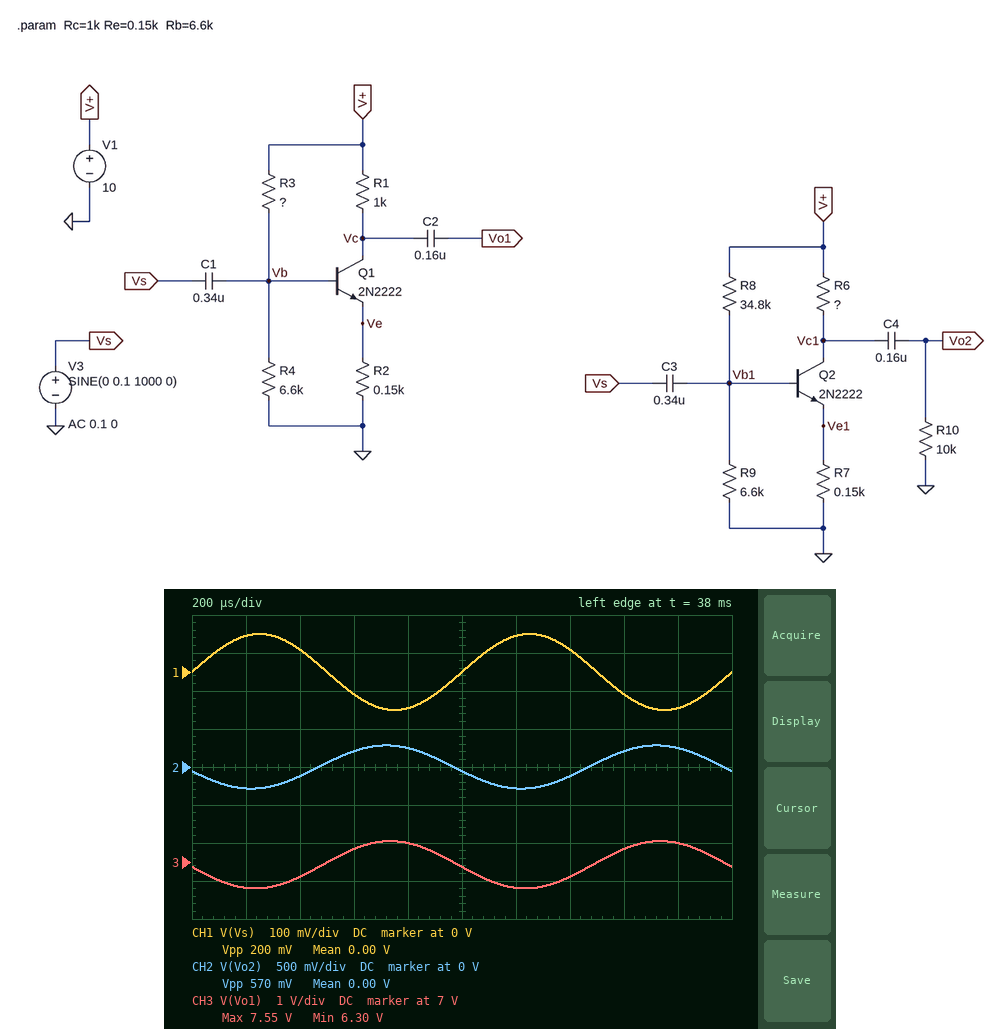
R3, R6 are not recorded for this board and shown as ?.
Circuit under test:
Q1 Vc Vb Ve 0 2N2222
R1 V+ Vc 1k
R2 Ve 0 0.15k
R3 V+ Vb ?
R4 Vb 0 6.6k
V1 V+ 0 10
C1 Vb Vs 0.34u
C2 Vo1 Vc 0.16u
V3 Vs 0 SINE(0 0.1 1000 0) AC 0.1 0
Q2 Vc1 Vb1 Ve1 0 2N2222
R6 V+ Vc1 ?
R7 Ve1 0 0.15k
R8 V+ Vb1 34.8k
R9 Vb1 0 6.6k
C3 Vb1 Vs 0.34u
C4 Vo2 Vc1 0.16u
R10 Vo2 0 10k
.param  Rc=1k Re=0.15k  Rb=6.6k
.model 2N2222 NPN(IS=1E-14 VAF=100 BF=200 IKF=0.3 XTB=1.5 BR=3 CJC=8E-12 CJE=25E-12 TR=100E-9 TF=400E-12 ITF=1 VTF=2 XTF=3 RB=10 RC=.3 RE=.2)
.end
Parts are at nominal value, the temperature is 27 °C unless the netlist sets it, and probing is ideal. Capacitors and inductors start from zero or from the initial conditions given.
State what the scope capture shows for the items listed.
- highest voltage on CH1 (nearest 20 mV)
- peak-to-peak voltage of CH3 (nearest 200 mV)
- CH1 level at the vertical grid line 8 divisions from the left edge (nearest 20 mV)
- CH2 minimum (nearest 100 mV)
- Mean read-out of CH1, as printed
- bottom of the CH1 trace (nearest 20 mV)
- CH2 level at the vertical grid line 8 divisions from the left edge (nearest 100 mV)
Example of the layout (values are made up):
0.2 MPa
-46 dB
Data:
100 mV
1.2 V
-60 mV
-300 mV
0.00 V
-100 mV
200 mV
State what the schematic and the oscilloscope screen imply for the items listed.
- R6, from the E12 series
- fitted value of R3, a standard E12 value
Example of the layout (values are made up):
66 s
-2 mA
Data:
470 Ω
47 kΩ
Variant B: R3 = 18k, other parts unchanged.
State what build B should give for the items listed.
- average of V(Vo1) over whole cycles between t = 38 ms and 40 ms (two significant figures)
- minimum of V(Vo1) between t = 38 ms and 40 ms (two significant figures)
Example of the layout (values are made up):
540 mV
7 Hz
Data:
1.5 V
1.4 V
